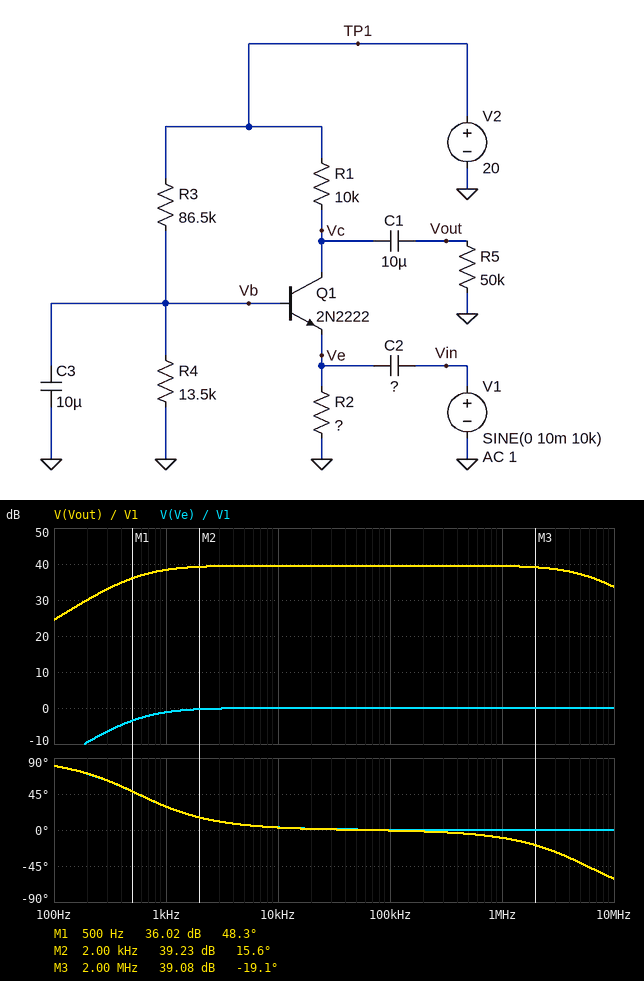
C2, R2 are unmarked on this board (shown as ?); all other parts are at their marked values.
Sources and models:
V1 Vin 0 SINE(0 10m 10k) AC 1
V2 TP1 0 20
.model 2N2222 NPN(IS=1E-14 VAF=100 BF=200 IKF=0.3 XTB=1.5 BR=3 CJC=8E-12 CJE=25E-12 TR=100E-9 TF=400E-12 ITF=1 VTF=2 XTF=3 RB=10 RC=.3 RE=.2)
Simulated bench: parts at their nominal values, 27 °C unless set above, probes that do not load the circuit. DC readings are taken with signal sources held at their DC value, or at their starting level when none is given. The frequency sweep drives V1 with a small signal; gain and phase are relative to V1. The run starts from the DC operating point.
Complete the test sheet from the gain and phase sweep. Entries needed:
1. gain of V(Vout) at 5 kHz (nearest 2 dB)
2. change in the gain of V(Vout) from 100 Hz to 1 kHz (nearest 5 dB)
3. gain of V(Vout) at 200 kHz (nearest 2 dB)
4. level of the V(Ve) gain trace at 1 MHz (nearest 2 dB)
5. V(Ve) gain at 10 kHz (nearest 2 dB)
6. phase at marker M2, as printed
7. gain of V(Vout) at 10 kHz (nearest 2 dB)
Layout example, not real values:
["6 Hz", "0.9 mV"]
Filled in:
["40 dB", "15 dB", "40 dB", "0 dB", "0 dB", "15.6 deg", "40 dB"]
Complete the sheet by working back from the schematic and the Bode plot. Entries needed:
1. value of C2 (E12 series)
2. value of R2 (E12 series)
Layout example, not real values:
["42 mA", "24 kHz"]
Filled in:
["3.3 µF", "6.8 kΩ"]
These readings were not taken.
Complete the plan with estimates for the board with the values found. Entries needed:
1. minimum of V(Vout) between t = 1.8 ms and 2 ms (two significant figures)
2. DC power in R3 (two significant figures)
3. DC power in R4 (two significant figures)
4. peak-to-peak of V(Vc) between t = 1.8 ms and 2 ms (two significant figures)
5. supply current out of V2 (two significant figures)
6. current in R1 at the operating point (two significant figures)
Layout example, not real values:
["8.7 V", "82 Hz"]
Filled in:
["-1.0 V", "3.5 mW", "530 µW", "1.9 V", "500 µA", "300 µA"]
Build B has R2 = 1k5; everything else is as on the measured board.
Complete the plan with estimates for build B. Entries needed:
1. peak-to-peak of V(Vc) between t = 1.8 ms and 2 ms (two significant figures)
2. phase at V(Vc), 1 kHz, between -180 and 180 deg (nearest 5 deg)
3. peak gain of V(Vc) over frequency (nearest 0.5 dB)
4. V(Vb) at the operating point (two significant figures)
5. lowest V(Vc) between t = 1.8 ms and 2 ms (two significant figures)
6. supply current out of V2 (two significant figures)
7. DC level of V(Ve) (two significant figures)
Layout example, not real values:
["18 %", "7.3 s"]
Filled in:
["7.2 V", "65 deg", "51.5 dB", "2.6 V", "3.1 V", "1.5 mA", "2.0 V"]
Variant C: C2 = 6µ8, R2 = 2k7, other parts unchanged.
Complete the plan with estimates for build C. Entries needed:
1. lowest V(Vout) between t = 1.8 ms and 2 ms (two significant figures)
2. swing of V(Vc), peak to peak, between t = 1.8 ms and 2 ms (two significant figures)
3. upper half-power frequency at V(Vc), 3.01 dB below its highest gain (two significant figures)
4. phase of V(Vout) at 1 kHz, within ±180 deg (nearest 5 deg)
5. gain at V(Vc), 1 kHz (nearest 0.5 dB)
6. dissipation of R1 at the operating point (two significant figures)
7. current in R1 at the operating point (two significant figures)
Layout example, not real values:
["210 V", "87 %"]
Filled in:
["-2.4 V", "4.4 V", "4.7 MHz", "35 deg", "45.5 dB", "5.5 mW", "740 µA"]
